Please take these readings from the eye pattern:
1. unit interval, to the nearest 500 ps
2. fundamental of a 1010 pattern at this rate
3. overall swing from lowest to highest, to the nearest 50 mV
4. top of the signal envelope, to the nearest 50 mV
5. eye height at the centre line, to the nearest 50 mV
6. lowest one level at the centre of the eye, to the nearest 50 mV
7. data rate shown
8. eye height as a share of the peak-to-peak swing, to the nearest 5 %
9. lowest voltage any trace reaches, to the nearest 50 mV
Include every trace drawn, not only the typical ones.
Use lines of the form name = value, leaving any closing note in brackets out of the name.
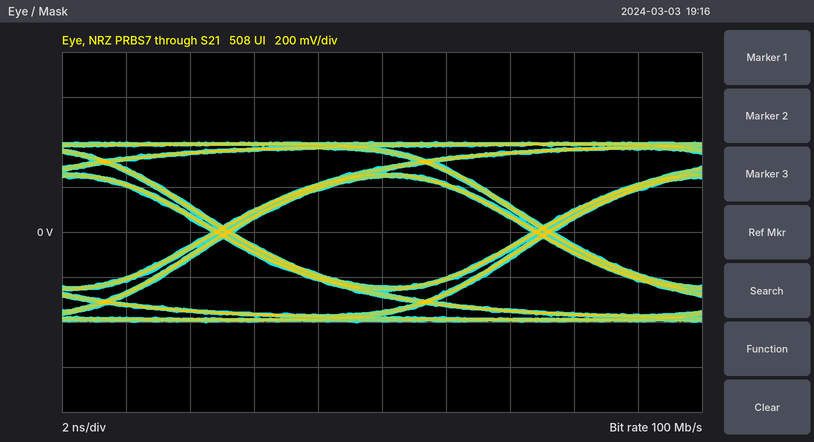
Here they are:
unit interval, to the nearest 500 ps = 10.0 ns
fundamental of a 1010 pattern at this rate = 50 MHz
overall swing from lowest to highest, to the nearest 50 mV = 800 mV
top of the signal envelope, to the nearest 50 mV = 400 mV
eye height at the centre line, to the nearest 50 mV = 500 mV
lowest one level at the centre of the eye, to the nearest 50 mV = 250 mV
data rate shown = 100 Mb/s
eye height as a share of the peak-to-peak swing, to the nearest 5 % = 60 %
lowest voltage any trace reaches, to the nearest 50 mV = -400 mV
